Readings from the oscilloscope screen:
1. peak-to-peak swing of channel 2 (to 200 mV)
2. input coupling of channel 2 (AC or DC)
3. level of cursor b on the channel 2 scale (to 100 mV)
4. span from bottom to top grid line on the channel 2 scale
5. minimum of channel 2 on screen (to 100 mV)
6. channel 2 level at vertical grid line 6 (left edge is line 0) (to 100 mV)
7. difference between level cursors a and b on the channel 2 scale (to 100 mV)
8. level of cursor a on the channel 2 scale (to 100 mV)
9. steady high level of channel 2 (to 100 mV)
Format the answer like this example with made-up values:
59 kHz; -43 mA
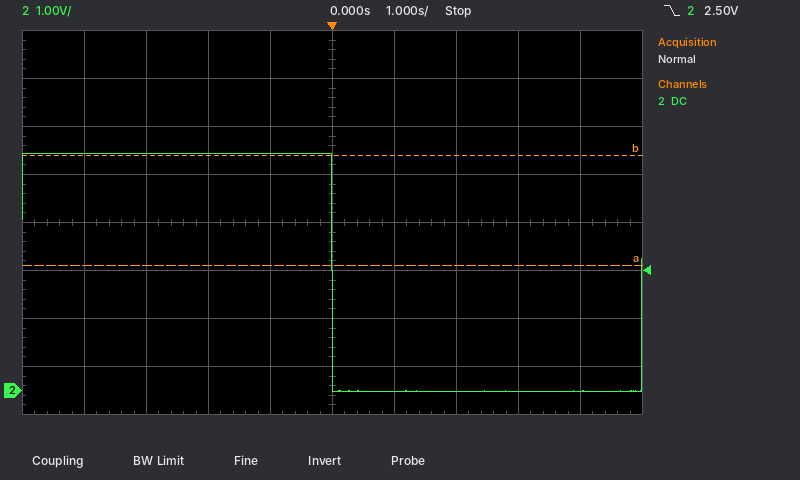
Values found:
5.0 V; DC; 4.9 V; 8 V; 0.0 V; 0.0 V; 2.3 V; 2.6 V; 4.9 V
